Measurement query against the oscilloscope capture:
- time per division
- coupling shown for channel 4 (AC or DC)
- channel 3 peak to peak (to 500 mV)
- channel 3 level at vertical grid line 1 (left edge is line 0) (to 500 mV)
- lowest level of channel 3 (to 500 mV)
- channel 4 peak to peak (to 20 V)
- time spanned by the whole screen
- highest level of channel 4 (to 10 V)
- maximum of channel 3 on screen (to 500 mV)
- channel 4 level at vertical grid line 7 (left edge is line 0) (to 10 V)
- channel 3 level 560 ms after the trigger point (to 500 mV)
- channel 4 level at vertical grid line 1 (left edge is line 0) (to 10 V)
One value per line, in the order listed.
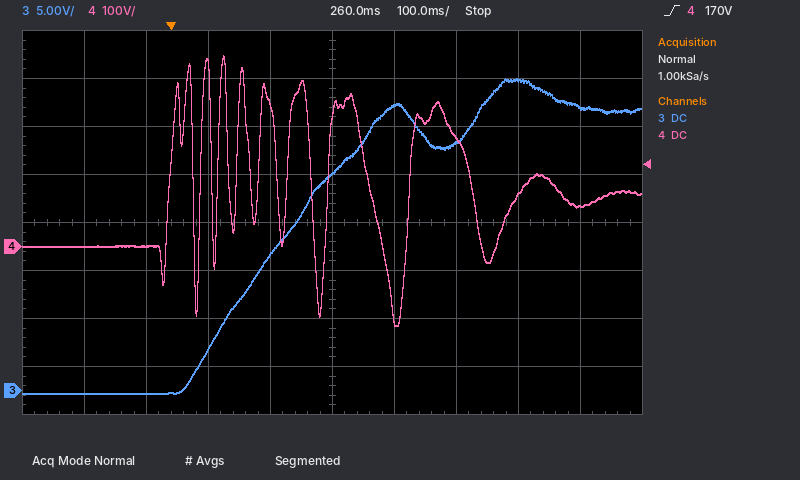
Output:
100 ms
DC
33.0 V
-500 mV
-500 mV
560 V
1 s
400 V
32.5 V
230 V
32.5 V
0 V
